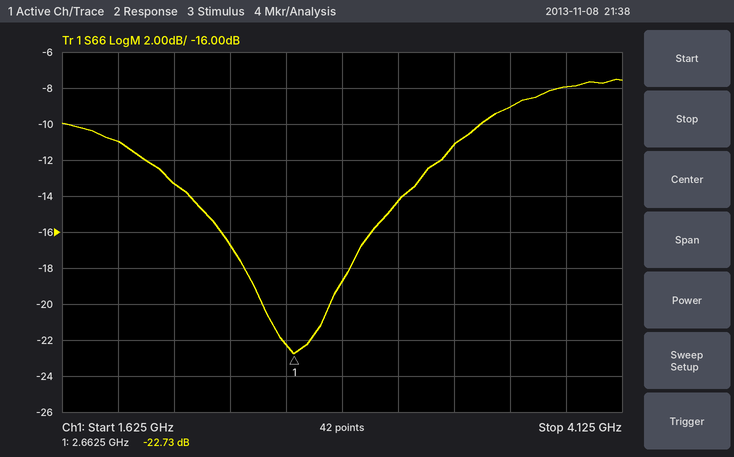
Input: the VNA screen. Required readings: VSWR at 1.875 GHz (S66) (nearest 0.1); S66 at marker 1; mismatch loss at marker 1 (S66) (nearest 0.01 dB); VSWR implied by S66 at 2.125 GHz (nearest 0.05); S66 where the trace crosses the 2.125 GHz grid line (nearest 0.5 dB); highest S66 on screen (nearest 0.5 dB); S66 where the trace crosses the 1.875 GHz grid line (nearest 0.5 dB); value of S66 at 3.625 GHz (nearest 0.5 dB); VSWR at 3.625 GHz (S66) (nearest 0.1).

1.8
-22.73 dB
0.02 dB
1.55
-13.5 dB
-7.5 dB
-11.0 dB
-9.0 dB
2.1
